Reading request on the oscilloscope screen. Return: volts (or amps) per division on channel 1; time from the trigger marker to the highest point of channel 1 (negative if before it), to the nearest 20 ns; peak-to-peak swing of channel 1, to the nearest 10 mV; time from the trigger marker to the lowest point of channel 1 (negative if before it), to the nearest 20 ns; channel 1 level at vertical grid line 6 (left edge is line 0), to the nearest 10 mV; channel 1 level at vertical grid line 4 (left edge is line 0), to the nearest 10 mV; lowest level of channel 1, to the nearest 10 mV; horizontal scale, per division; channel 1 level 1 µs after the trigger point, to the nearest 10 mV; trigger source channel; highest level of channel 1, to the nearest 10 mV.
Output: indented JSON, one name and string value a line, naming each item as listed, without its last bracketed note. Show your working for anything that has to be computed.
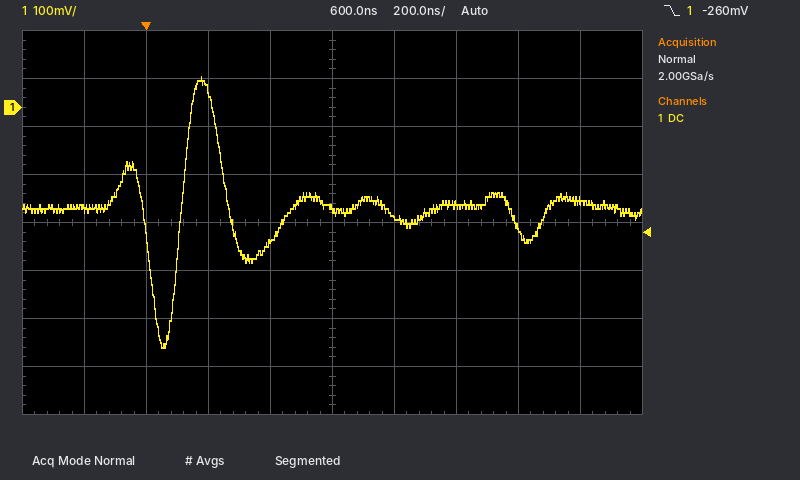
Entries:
{
  "volts (or amps) per division on channel 1": "100 mV",
  "time from the trigger marker to the highest point of channel 1 (negative if before it), to the nearest 20 ns": "+180 ns",
  "peak-to-peak swing of channel 1, to the nearest 10 mV": "60 mV − (-500 mV) = 560 mV",
  "time from the trigger marker to the lowest point of channel 1 (negative if before it), to the nearest 20 ns": "+60 ns",
  "channel 1 level at vertical grid line 6 (left edge is line 0), to the nearest 10 mV": "-230 mV",
  "channel 1 level at vertical grid line 4 (left edge is line 0), to the nearest 10 mV": "-280 mV",
  "lowest level of channel 1, to the nearest 10 mV": "-500 mV",
  "horizontal scale, per division": "200 ns",
  "channel 1 level 1 µs after the trigger point, to the nearest 10 mV": "-200 mV",
  "trigger source channel": "channel 1",
  "highest level of channel 1, to the nearest 10 mV": "60 mV"
}
